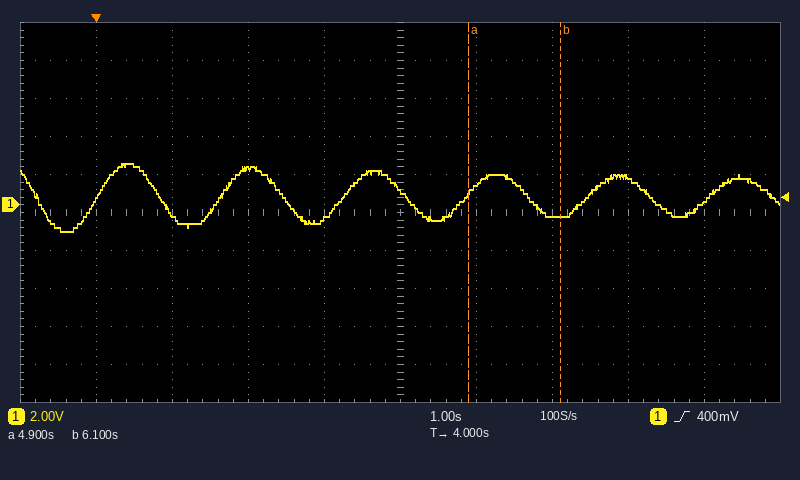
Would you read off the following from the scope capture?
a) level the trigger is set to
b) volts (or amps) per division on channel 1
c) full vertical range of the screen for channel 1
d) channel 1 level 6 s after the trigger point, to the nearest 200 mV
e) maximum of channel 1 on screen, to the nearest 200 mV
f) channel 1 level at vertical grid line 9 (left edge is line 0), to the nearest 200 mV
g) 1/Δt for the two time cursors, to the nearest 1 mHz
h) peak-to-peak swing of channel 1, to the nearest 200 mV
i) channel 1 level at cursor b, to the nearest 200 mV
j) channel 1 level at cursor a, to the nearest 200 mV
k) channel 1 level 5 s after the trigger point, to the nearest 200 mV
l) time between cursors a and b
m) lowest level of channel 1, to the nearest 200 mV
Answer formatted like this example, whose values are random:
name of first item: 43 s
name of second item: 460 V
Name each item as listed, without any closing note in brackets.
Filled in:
level the trigger is set to: 400 mV
volts (or amps) per division on channel 1: 2 V
full vertical range of the screen for channel 1: 20 V
channel 1 level 6 s after the trigger point, to the nearest 200 mV: -600 mV
maximum of channel 1 on screen, to the nearest 200 mV: 2.2 V
channel 1 level at vertical grid line 9 (left edge is line 0), to the nearest 200 mV: 200 mV
1/Δt for the two time cursors, to the nearest 1 mHz: 833 mHz
peak-to-peak swing of channel 1, to the nearest 200 mV: 3.6 V
channel 1 level at cursor b, to the nearest 200 mV: -600 mV
channel 1 level at cursor a, to the nearest 200 mV: 600 mV
channel 1 level 5 s after the trigger point, to the nearest 200 mV: 1.0 V
time between cursors a and b: 1.2 s
lowest level of channel 1, to the nearest 200 mV: -1.4 V
